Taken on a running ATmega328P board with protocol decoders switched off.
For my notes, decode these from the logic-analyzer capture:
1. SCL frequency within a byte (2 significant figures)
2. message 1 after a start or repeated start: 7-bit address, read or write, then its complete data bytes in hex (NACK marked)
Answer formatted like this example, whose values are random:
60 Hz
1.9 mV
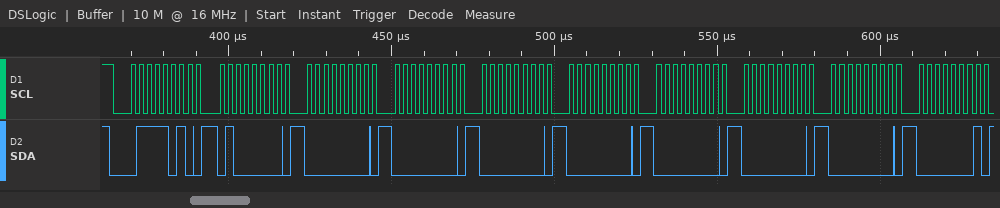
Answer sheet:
400 kHz
0x3D write: 40 00 00 00 00 00 00 00 01
